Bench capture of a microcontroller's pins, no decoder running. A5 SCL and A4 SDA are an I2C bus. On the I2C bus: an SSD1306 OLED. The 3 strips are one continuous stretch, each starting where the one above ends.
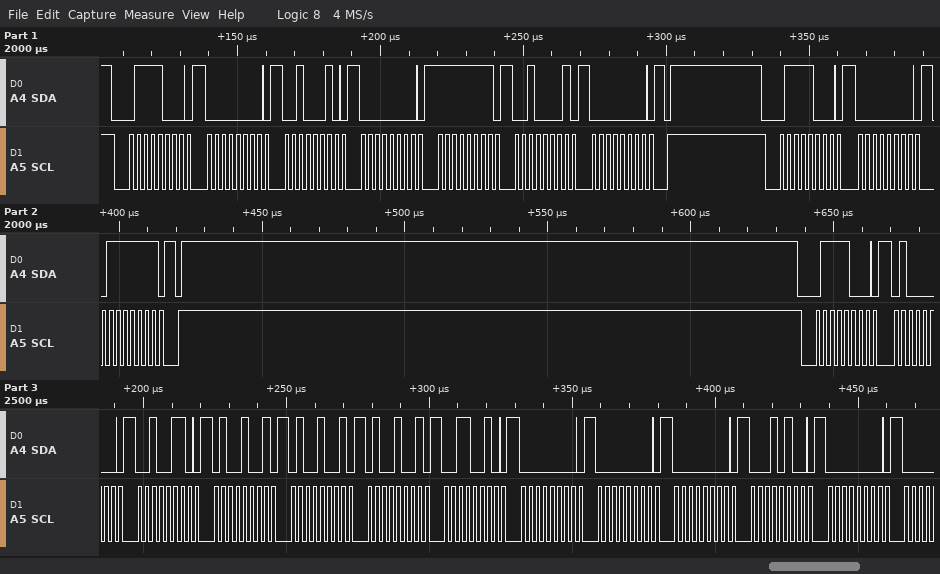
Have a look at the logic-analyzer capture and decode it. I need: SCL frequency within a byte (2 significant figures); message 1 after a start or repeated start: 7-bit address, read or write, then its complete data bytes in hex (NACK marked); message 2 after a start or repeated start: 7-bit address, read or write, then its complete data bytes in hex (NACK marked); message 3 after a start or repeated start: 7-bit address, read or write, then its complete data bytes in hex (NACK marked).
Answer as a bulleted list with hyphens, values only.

- 400 kHz
- 0x3C write: 00 22 00 FF 21 00
- 0x3C write: 00 7F
- 0x3C write: 40 26 49 49 49 32 00 00 00 14 00
